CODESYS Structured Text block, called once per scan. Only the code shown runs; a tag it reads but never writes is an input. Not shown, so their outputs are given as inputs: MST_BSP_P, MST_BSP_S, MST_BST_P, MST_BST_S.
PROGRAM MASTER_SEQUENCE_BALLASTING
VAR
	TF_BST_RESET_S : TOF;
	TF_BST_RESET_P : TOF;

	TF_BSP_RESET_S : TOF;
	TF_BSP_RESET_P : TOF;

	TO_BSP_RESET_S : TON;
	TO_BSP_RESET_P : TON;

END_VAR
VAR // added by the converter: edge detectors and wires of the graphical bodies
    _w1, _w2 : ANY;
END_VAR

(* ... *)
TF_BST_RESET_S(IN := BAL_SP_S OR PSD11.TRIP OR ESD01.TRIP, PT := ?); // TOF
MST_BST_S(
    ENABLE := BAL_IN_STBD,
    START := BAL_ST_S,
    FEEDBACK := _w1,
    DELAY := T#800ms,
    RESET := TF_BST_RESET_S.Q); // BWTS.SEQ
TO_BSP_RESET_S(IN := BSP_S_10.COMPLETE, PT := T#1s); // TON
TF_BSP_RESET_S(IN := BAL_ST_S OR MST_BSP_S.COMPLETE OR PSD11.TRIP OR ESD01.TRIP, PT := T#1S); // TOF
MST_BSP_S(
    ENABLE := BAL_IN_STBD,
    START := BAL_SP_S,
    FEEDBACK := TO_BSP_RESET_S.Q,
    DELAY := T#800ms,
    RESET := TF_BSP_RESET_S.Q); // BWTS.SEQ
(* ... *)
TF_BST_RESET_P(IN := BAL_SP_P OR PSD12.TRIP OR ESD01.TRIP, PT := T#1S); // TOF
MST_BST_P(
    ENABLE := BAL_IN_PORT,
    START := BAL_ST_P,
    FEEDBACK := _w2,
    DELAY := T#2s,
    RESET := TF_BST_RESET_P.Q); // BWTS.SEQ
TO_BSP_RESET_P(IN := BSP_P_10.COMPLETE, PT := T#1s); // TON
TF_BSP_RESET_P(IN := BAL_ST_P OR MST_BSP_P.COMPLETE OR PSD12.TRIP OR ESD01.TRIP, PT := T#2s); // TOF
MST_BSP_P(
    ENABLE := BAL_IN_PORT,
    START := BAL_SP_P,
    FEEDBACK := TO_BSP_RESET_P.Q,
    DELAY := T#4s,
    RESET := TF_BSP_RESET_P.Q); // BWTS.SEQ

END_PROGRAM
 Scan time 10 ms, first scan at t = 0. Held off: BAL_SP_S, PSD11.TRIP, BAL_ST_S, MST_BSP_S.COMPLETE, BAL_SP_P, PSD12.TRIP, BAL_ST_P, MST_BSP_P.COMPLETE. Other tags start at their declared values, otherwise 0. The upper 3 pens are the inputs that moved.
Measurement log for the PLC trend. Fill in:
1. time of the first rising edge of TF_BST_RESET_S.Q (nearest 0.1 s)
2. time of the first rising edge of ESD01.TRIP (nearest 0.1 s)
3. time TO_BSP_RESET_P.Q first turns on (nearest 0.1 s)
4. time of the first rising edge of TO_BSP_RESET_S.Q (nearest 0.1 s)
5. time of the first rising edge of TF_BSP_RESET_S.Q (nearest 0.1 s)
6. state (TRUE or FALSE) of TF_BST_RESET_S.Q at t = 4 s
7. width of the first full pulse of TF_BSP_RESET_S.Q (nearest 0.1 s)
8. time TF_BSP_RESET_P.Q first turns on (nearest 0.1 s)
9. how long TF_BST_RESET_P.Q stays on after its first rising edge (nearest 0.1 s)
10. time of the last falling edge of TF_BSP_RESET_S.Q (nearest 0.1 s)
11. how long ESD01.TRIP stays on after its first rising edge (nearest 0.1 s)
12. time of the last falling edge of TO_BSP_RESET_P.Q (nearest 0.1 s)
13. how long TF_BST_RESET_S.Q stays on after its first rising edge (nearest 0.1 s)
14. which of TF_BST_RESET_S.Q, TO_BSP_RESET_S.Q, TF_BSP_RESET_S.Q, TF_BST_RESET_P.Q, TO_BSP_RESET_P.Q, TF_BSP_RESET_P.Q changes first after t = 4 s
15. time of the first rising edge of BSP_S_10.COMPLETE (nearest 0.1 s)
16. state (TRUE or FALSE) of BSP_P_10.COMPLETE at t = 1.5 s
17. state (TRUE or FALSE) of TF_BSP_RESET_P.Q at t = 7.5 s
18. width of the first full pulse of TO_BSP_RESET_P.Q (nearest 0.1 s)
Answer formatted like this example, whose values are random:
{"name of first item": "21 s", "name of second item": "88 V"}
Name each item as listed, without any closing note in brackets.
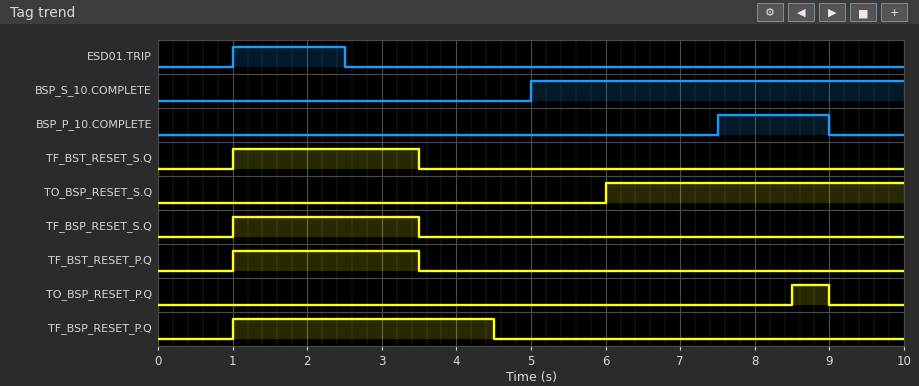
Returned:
{"time of the first rising edge of TF_BST_RESET_S.Q": "1.0 s", "time of the first rising edge of ESD01.TRIP": "1.0 s", "time TO_BSP_RESET_P.Q first turns on": "8.5 s", "time of the first rising edge of TO_BSP_RESET_S.Q": "6.0 s", "time of the first rising edge of TF_BSP_RESET_S.Q": "1.0 s", "state (TRUE or FALSE) of TF_BST_RESET_S.Q at t = 4 s": "FALSE", "width of the first full pulse of TF_BSP_RESET_S.Q": "2.5 s", "time TF_BSP_RESET_P.Q first turns on": "1.0 s", "how long TF_BST_RESET_P.Q stays on after its first rising edge": "2.5 s", "time of the last falling edge of TF_BSP_RESET_S.Q": "3.5 s", "how long ESD01.TRIP stays on after its first rising edge": "1.5 s", "time of the last falling edge of TO_BSP_RESET_P.Q": "9.0 s", "how long TF_BST_RESET_S.Q stays on after its first rising edge": "2.5 s", "which of TF_BST_RESET_S.Q, TO_BSP_RESET_S.Q, TF_BSP_RESET_S.Q, TF_BST_RESET_P.Q, TO_BSP_RESET_P.Q, TF_BSP_RESET_P.Q changes first after t = 4 s": "TF_BSP_RESET_P.Q", "time of the first rising edge of BSP_S_10.COMPLETE": "5.0 s", "state (TRUE or FALSE) of BSP_P_10.COMPLETE at t = 1.5 s": "FALSE", "state (TRUE or FALSE) of TF_BSP_RESET_P.Q at t = 7.5 s": "FALSE", "width of the first full pulse of TO_BSP_RESET_P.Q": "0.5 s"}
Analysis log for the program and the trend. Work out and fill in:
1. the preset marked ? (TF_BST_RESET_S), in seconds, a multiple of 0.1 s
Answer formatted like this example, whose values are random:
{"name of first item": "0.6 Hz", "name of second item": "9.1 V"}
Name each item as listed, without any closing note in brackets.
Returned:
{"the preset marked ? (TF_BST_RESET_S), in seconds, a multiple of 0.1 s": "1.0 s"}
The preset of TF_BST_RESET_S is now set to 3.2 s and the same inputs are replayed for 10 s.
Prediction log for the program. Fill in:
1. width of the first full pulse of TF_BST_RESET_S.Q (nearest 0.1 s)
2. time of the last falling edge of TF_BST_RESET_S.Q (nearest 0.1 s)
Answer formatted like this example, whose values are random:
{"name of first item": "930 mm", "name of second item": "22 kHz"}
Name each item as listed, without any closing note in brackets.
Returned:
{"width of the first full pulse of TF_BST_RESET_S.Q": "4.7 s", "time of the last falling edge of TF_BST_RESET_S.Q": "5.7 s"}
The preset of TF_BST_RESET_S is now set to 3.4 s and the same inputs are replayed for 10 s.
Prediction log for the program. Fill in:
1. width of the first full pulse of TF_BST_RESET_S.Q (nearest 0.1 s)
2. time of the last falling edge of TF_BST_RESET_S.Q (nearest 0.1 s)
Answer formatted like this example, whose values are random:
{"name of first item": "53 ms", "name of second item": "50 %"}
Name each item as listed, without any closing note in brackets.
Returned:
{"width of the first full pulse of TF_BST_RESET_S.Q": "4.9 s", "time of the last falling edge of TF_BST_RESET_S.Q": "5.9 s"}
